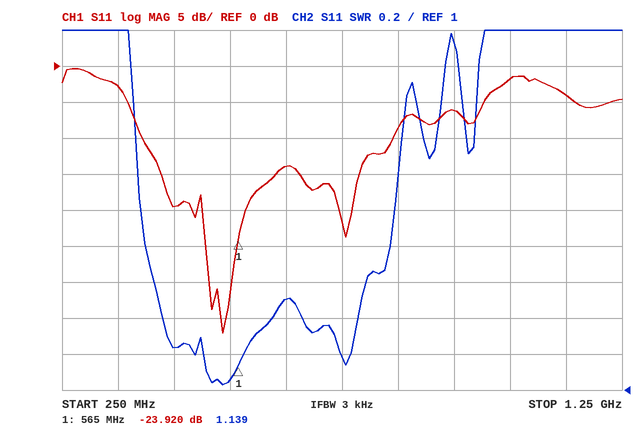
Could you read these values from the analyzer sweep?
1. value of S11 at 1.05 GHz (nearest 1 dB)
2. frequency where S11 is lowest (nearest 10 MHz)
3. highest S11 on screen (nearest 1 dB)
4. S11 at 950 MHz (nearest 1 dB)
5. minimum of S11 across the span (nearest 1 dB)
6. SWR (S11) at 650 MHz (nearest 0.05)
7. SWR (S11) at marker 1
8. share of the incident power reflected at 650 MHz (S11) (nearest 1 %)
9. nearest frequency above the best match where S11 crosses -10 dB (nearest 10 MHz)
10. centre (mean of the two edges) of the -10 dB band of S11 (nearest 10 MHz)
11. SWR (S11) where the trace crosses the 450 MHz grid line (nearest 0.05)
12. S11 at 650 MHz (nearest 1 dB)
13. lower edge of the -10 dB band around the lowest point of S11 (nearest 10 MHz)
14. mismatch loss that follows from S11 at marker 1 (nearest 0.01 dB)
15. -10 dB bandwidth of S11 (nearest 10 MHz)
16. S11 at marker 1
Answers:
-2 dB
540 MHz
0 dB
-6 dB
-37 dB
1.50
1.139
4 %
840 MHz
620 MHz
1.25
-14 dB
390 MHz
0.02 dB
450 MHz
-23.920 dB
